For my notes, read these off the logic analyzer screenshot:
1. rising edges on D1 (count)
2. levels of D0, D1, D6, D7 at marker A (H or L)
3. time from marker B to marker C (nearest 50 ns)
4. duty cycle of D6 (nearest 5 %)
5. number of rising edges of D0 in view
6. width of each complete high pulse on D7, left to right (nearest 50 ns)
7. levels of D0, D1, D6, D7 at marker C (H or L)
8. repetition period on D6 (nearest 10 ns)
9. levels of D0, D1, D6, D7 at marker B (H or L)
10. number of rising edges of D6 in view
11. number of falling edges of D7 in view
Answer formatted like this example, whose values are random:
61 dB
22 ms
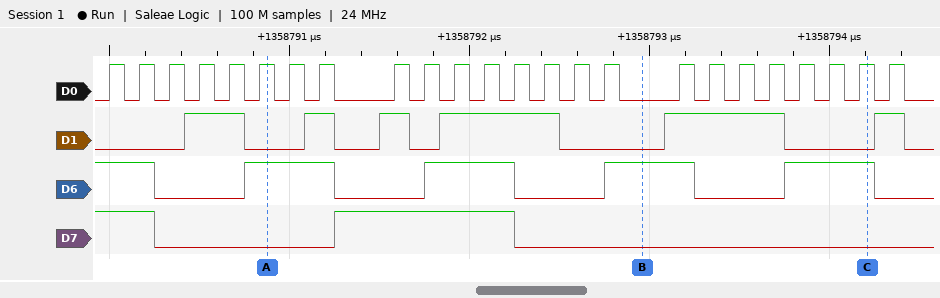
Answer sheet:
6
D0=H, D1=L, D6=H, D7=L
1250 ns
50 %
24
1000 ns
D0=H, D1=L, D6=H, D7=L
1000 ns
D0=L, D1=L, D6=H, D7=L
4
2
